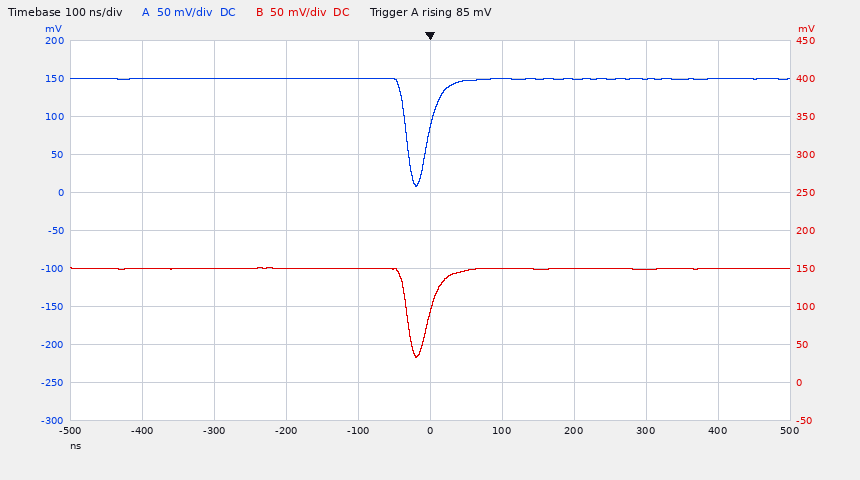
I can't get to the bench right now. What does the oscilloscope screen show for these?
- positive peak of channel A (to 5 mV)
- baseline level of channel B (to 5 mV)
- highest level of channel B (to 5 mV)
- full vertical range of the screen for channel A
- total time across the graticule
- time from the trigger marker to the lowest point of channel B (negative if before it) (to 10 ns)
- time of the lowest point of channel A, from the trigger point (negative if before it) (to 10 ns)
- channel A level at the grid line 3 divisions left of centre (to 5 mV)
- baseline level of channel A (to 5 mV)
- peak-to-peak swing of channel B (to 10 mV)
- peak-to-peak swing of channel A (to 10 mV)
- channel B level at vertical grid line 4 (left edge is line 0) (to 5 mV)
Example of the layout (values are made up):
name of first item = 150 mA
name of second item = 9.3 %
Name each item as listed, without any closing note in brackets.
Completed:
positive peak of channel A = 150 mV
baseline level of channel B = 150 mV
highest level of channel B = 150 mV
full vertical range of the screen for channel A = 500 mV
total time across the graticule = 1 µs
time from the trigger marker to the lowest point of channel B (negative if before it) = -20 ns
time of the lowest point of channel A, from the trigger point (negative if before it) = -20 ns
channel A level at the grid line 3 divisions left of centre = 150 mV
baseline level of channel A = 150 mV
peak-to-peak swing of channel B = 120 mV
peak-to-peak swing of channel A = 140 mV
channel B level at vertical grid line 4 (left edge is line 0) = 150 mV
